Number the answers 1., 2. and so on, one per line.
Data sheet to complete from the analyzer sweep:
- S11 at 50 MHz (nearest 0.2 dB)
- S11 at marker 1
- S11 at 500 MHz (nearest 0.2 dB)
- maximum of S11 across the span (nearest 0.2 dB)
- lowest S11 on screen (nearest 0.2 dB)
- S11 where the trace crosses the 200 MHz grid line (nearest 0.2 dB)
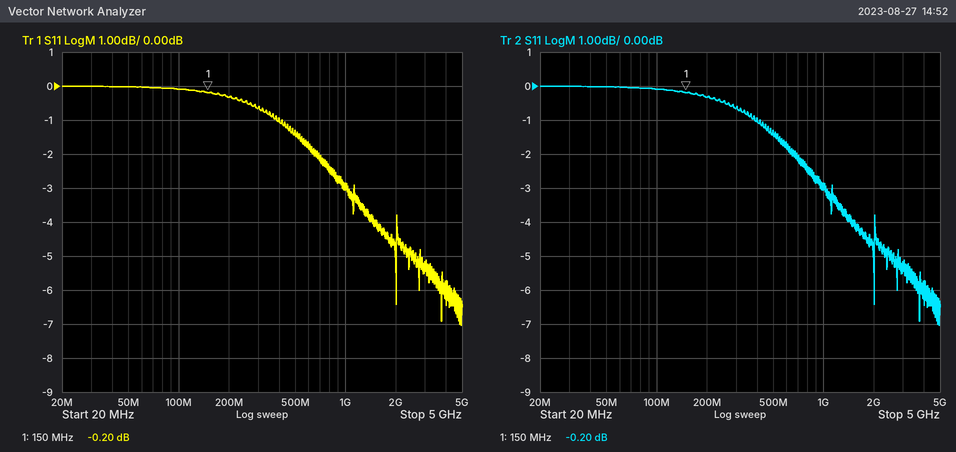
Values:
1. 0.0 dB
2. -0.20 dB
3. -1.4 dB
4. 0.0 dB
5. -7.0 dB
6. -0.4 dB
